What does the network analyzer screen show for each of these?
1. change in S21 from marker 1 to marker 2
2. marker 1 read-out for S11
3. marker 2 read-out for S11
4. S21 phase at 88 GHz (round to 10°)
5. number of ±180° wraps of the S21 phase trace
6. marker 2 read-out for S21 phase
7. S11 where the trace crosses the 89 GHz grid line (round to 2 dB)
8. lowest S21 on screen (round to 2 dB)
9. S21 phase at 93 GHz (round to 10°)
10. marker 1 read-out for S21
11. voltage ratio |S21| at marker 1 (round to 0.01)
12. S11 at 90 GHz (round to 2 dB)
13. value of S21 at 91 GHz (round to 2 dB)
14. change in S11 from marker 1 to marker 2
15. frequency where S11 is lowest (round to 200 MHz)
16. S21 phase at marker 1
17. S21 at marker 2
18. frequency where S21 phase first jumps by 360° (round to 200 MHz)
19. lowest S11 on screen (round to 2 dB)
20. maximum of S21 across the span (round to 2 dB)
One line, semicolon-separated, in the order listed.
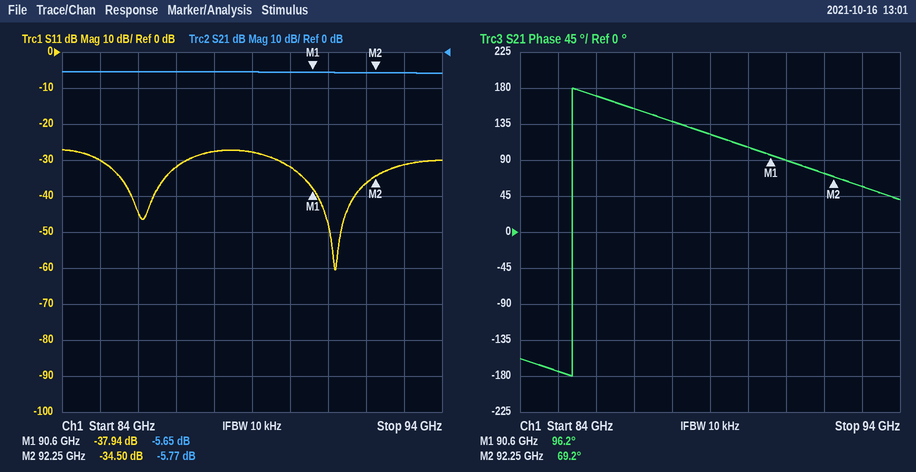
-0.12 dB; -37.94 dB; -34.50 dB; 140°; 1; 69.2°; -28 dB; -6 dB; 60°; -5.65 dB; 0.52; -32 dB; -6 dB; 3.44 dB; 91.2 GHz; 96.2°; -5.77 dB; 85.4 GHz; -60 dB; -6 dB
